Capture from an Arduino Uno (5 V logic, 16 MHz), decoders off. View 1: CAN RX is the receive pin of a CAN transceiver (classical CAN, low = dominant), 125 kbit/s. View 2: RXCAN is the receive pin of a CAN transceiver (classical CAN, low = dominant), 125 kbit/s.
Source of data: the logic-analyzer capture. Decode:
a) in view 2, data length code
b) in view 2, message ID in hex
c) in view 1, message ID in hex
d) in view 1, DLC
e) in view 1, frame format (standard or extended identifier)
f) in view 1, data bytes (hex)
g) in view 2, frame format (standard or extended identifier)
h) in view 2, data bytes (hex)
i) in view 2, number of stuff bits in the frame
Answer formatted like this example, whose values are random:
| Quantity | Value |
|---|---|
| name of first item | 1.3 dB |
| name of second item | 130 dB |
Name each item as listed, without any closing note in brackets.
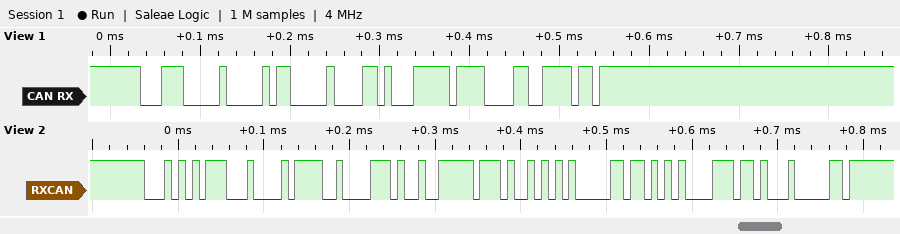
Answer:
| Quantity | Value |
|---|---|
| in view 2, data length code | 8 |
| in view 2, message ID in hex | 0x157 |
| in view 1, message ID in hex | 0x1C0 |
| in view 1, DLC | 3 |
| in view 1, frame format | standard |
| in view 1, data bytes | 00 68 FF |
| in view 2, frame format | standard |
| in view 2, data bytes | 5E 43 A4 FF 4A A0 B5 43 |
| in view 2, number of stuff bits in the frame | 3 |
